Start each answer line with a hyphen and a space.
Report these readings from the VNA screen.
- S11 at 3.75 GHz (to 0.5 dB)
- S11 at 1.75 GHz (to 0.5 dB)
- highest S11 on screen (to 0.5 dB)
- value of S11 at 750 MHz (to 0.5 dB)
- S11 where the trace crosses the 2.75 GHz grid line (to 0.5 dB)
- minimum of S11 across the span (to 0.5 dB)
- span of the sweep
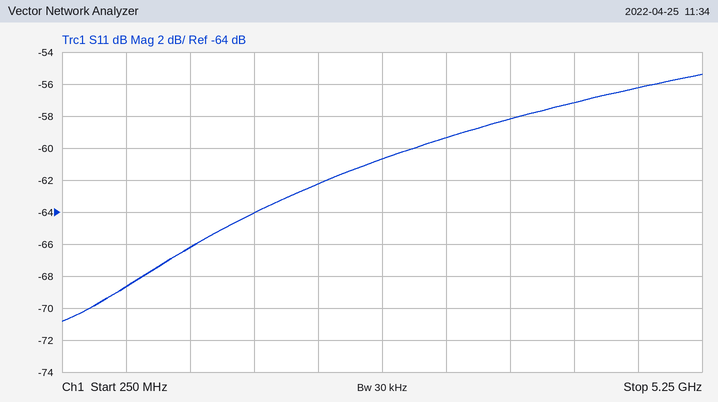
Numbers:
- -58.0 dB
- -64.0 dB
- -55.5 dB
- -68.5 dB
- -60.5 dB
- -71.0 dB
- 5 GHz
